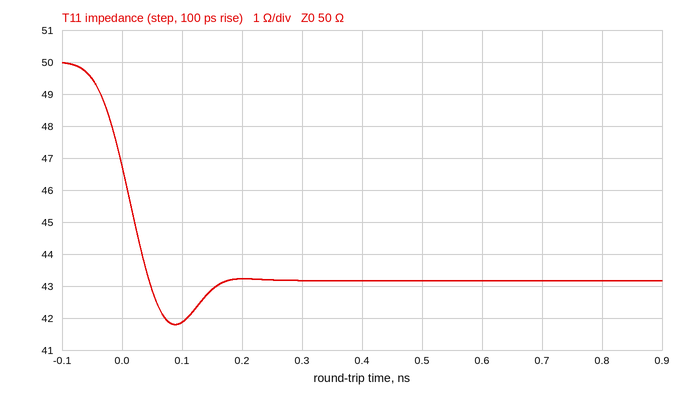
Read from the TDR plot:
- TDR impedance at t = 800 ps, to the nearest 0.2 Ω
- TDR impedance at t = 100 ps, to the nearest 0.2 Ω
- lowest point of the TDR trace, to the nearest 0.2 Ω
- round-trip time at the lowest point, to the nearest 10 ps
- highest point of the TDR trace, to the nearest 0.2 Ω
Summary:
43.2 Ω
41.8 Ω
41.8 Ω
90 ps
50.0 Ω
